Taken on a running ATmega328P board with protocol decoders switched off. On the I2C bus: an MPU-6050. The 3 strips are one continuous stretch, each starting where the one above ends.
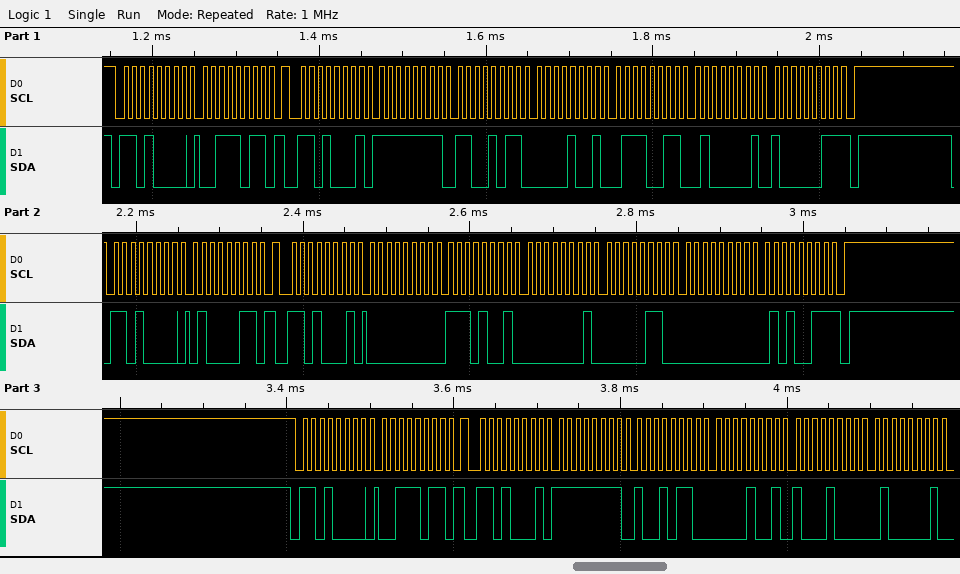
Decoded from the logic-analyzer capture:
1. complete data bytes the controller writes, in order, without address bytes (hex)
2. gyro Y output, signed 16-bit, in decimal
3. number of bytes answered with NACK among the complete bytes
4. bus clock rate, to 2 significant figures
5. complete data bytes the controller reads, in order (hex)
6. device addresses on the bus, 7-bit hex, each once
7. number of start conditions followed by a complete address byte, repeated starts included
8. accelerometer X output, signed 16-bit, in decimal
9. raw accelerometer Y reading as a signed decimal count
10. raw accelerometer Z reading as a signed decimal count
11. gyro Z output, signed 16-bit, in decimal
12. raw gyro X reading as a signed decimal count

3B 43 3B
262
2
100 kHz
FF CB 09 73 41 83 00 E9 01 06 00 53 FF 96 09 88 41
0x68
6
-53
2419
16771
83
233
